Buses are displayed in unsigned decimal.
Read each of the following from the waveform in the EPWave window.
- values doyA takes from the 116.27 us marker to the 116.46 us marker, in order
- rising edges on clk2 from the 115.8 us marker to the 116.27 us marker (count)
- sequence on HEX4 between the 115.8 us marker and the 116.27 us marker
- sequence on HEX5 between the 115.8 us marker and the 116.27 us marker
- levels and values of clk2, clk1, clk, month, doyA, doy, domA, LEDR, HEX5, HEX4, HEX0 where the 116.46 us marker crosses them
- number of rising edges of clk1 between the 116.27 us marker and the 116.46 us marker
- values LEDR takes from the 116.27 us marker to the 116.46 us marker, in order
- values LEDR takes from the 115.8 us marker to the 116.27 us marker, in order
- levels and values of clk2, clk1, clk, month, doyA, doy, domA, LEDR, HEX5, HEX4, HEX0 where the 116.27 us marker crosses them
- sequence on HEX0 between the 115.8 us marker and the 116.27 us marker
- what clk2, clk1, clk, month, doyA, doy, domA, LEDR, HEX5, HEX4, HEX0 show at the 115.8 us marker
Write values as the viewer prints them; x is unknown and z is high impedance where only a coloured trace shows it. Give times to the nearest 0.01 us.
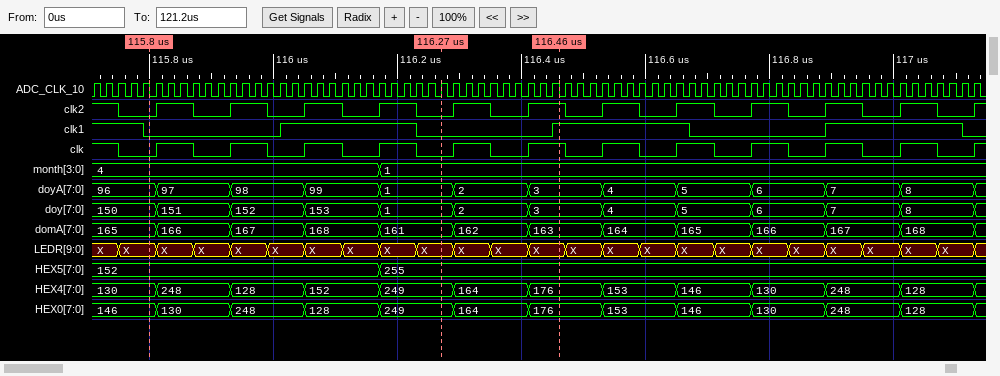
1, 2, 3
4
130, 248, 128, 152, 249
152, 255
clk2=1, clk1=1, clk=1, month=1, doyA=3, doy=3, domA=163, LEDR=X, HEX5=255, HEX4=176, HEX0=176
1
X, X, X, X
X, X, X, X, X, X, X, X, X
clk2=0, clk1=0, clk=0, month=1, doyA=1, doy=1, domA=161, LEDR=X, HEX5=255, HEX4=249, HEX0=249
146, 130, 248, 128, 249
clk2=0, clk1=0, clk=0, month=4, doyA=96, doy=150, domA=165, LEDR=X, HEX5=152, HEX4=130, HEX0=146
